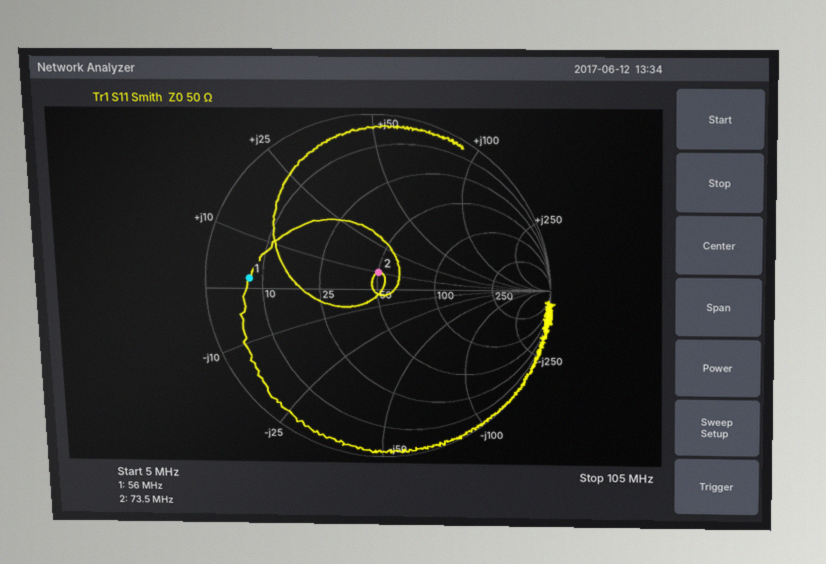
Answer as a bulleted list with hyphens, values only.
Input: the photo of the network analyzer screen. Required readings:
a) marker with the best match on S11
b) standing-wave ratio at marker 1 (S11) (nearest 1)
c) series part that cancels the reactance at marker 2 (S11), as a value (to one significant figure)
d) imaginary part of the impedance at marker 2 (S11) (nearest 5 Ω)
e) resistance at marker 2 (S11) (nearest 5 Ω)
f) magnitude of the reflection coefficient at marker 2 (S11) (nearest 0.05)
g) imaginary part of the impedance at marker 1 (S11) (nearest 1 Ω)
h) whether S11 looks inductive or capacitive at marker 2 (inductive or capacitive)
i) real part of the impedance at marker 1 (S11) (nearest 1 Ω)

- marker 2
- 7
- 200 pF
- +10 Ω
- 50 Ω
- 0.10
- +2 Ω
- inductive
- 7 Ω
